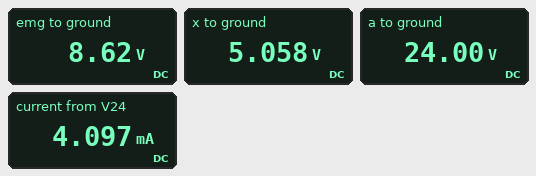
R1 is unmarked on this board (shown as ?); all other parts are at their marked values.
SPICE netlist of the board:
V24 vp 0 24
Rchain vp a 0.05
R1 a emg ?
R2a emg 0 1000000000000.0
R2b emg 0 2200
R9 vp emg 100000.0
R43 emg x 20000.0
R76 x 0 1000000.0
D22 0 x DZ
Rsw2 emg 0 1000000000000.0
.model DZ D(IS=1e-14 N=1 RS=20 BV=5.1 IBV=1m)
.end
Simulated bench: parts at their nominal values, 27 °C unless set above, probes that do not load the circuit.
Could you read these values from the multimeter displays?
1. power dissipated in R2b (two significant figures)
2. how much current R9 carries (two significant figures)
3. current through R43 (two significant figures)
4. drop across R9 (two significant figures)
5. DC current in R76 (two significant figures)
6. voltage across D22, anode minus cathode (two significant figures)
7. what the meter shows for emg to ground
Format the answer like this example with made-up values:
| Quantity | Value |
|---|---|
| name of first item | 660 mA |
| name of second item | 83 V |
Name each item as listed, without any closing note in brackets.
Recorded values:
| Quantity | Value |
|---|---|
| power dissipated in R2b | 34 mW |
| how much current R9 carries | 150 µA |
| current through R43 | 180 µA |
| drop across R9 | 15 V |
| DC current in R76 | 5.1 µA |
| voltage across D22, anode minus cathode | -5.1 V |
| what the meter shows for emg to ground | 8.62 V |
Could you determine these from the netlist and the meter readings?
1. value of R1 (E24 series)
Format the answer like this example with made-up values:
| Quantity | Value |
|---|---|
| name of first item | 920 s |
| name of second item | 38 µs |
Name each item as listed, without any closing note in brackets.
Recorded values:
| Quantity | Value |
|---|---|
| value of R1 | 3.9 kΩ |
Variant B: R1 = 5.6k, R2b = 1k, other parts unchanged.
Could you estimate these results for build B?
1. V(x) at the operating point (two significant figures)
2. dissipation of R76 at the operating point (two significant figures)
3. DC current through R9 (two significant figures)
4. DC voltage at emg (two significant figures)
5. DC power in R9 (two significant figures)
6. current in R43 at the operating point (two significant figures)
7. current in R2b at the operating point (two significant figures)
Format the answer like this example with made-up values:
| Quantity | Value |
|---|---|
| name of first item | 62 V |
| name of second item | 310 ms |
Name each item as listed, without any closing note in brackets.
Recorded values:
| Quantity | Value |
|---|---|
| V(x) at the operating point | 3.7 V |
| dissipation of R76 at the operating point | 14 µW |
| DC current through R9 | 200 µA |
| DC voltage at emg | 3.8 V |
| DC power in R9 | 4.1 mW |
| current in R43 at the operating point | 3.7 µA |
| current in R2b at the operating point | 3.8 mA |
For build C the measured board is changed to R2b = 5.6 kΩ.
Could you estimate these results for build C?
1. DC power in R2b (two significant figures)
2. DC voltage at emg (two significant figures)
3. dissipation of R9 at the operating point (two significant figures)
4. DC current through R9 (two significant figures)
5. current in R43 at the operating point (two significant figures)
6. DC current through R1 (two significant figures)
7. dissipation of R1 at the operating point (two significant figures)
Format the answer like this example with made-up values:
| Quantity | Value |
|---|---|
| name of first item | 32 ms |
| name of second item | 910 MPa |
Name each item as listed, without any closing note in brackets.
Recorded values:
| Quantity | Value |
|---|---|
| DC power in R2b | 32 mW |
| DC voltage at emg | 13 V |
| dissipation of R9 at the operating point | 1.1 mW |
| DC current through R9 | 110 µA |
| current in R43 at the operating point | 420 µA |
| DC current through R1 | 2.7 mA |
| dissipation of R1 at the operating point | 29 mW |
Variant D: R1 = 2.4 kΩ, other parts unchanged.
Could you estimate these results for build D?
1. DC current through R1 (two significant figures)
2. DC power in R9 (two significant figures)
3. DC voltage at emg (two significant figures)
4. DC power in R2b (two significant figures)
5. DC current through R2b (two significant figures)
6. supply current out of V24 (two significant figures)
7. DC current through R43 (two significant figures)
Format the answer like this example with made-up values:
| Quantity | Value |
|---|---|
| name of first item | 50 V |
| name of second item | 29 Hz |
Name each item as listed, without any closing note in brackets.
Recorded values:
| Quantity | Value |
|---|---|
| DC current through R1 | 5.3 mA |
| DC power in R9 | 1.6 mW |
| DC voltage at emg | 11 V |
| DC power in R2b | 58 mW |
| DC current through R2b | 5.1 mA |
| supply current out of V24 | 5.4 mA |
| DC current through R43 | 310 µA |
